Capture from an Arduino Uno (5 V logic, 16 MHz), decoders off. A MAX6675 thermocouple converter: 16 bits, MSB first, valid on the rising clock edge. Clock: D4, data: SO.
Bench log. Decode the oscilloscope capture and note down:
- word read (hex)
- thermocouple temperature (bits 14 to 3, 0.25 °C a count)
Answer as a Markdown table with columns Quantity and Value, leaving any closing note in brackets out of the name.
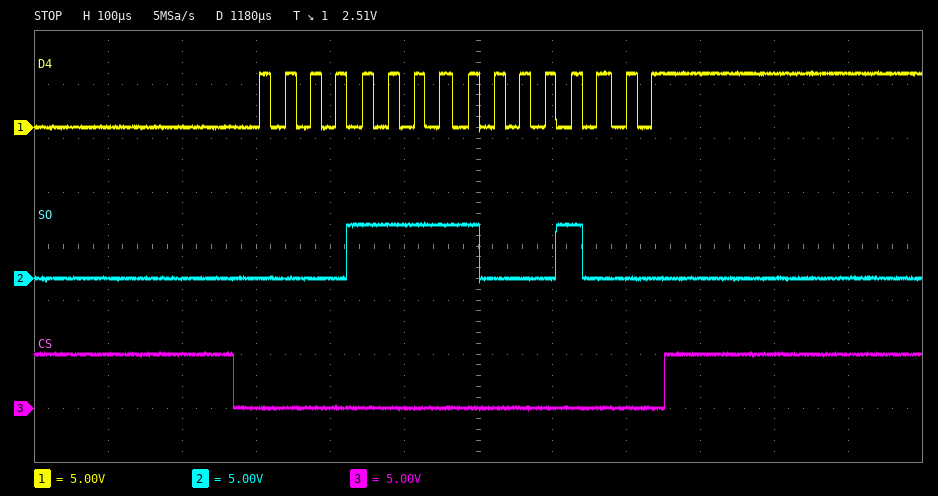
| Quantity | Value |
|---|---|
| word read | 0x0F88 |
| thermocouple temperature | 124.25 °C |
